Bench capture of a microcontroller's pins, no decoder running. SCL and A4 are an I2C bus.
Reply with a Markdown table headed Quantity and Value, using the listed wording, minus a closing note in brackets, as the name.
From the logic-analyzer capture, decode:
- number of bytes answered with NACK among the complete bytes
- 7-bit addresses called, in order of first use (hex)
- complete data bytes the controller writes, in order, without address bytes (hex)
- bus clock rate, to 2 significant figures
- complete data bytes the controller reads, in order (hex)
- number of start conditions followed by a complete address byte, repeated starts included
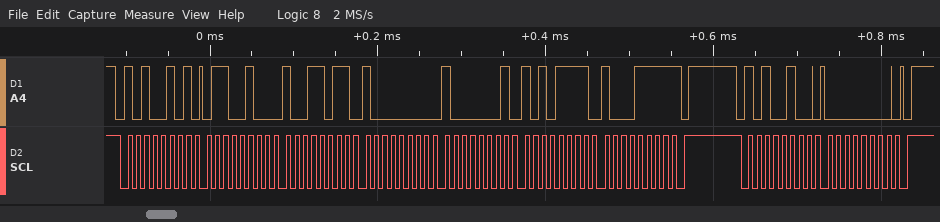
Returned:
| Quantity | Value |
|---|---|
| number of bytes answered with NACK among the complete bytes | 1 |
| 7-bit addresses called, in order of first use | 0x52 |
| complete data bytes the controller writes, in order, without address bytes | 00 |
| bus clock rate, to 2 significant figures | 100 kHz |
| complete data bytes the controller reads, in order | 64 9B 80 81 AF 8F |
| number of start conditions followed by a complete address byte, repeated starts included | 2 |
